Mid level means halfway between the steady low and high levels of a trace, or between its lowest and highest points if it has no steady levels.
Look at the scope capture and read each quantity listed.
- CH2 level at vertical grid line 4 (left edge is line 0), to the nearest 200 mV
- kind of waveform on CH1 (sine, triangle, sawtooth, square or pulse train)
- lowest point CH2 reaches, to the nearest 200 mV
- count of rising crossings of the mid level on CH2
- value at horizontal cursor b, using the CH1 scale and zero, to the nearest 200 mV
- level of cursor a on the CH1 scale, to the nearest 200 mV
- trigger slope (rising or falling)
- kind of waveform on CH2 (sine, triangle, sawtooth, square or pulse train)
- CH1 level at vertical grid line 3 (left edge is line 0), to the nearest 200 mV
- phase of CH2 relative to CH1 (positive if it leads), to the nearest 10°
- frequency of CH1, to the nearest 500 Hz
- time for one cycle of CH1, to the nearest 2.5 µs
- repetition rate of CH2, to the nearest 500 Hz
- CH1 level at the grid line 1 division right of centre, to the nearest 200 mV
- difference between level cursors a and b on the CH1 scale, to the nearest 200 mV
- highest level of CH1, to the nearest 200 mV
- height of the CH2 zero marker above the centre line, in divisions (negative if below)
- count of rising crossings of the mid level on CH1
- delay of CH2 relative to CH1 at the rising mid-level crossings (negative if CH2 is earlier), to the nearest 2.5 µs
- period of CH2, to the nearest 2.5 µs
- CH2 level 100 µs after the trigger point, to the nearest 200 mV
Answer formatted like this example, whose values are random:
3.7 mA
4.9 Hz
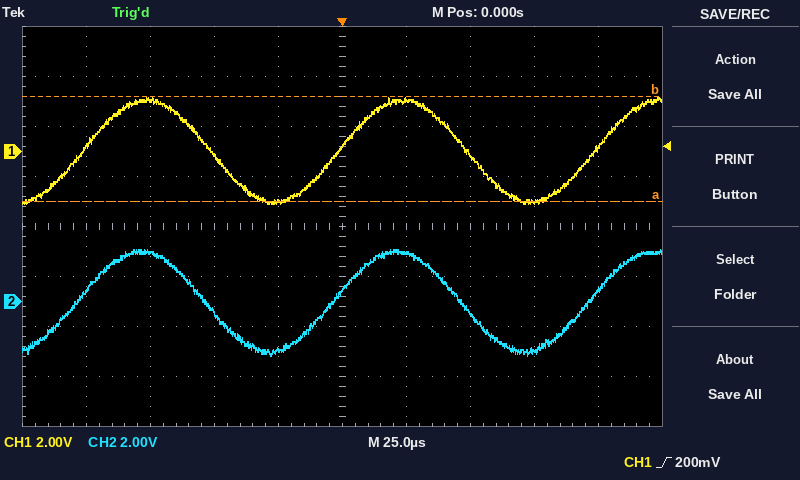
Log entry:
-2.0 V
sine
-2.2 V
3
2.2 V
-2.0 V
rising
sine
-200 mV
+10°
10.0 kHz
100.0 µs
10.0 kHz
2.0 V
4.2 V
2.2 V
-1.5 div
3
-2.5 µs
100.0 µs
400 mV
